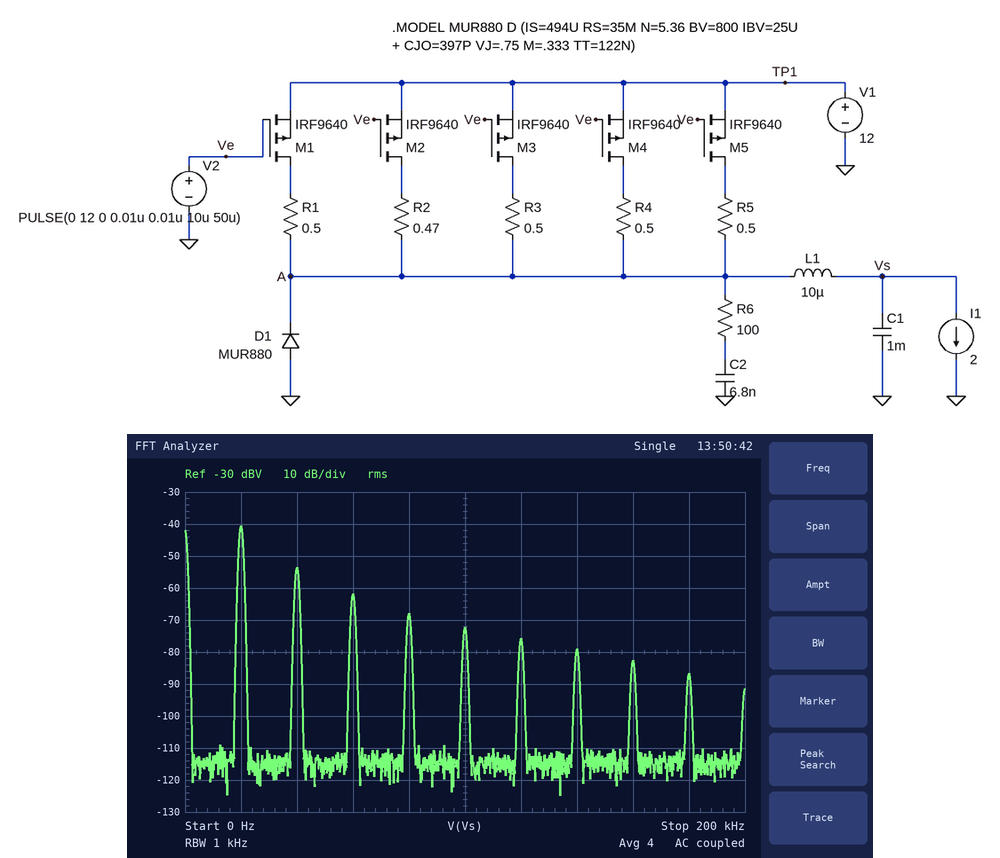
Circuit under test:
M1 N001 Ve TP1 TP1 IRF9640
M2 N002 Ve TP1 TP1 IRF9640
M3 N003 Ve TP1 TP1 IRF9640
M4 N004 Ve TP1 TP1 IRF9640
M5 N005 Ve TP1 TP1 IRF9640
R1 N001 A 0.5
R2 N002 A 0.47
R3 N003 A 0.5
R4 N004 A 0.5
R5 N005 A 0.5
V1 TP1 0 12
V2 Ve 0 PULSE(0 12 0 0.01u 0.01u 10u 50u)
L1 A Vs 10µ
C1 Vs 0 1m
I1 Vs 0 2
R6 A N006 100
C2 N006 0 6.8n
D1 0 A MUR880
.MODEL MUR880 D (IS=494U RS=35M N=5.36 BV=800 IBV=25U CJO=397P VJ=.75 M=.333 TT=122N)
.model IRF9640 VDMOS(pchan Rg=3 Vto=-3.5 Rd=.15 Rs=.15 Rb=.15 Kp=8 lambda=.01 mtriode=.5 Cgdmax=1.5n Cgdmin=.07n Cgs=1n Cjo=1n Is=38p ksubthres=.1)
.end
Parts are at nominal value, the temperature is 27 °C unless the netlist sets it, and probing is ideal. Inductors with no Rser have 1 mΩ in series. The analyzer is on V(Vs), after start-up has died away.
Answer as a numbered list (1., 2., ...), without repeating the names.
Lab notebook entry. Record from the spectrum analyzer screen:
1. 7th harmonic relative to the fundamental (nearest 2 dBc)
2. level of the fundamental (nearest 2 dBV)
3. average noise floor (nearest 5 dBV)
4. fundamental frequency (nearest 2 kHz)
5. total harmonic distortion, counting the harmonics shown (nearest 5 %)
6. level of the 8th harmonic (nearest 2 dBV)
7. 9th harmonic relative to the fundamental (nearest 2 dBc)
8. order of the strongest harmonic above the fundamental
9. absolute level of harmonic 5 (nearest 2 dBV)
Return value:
1. -38 dBc
2. -40 dBV
3. -115 dBV
4. 20 kHz
5. 25 %
6. -82 dBV
7. -46 dBc
8. 2
9. -72 dBV
